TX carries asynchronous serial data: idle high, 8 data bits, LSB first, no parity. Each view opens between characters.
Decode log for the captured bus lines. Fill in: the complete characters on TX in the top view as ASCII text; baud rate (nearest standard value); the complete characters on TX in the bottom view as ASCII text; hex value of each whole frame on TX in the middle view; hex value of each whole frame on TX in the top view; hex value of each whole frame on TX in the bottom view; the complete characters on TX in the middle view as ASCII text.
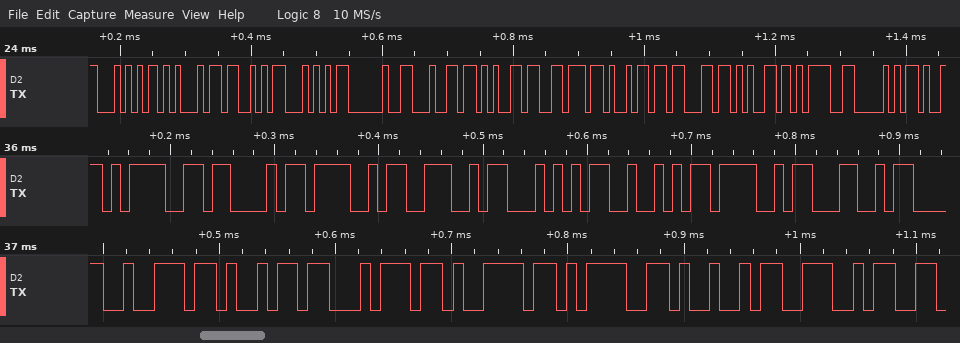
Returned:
"TEST device=P"
115200 baud
"rity=IN"
3D, 43, 4F, 4E, 54, 52, 4F, 4C
54, 45, 53, 54, 20, 64, 65, 76, 69, 63, 65, 3D, 50
72, 69, 74, 79, 3D, 49, 4E
"=CONTROL"
